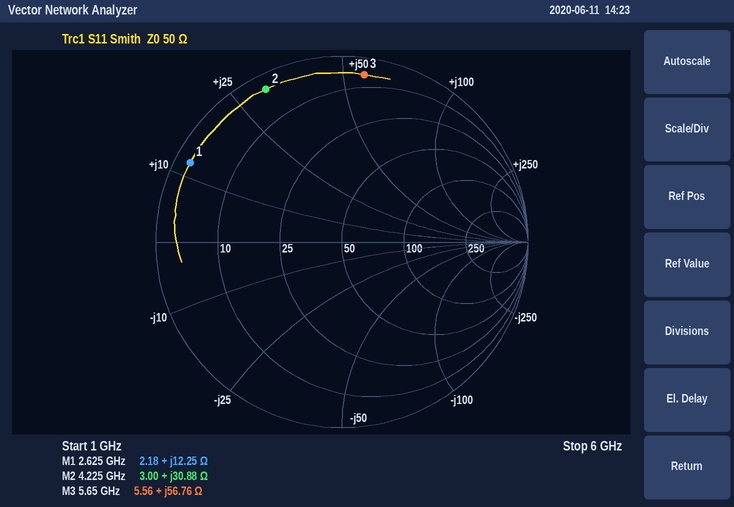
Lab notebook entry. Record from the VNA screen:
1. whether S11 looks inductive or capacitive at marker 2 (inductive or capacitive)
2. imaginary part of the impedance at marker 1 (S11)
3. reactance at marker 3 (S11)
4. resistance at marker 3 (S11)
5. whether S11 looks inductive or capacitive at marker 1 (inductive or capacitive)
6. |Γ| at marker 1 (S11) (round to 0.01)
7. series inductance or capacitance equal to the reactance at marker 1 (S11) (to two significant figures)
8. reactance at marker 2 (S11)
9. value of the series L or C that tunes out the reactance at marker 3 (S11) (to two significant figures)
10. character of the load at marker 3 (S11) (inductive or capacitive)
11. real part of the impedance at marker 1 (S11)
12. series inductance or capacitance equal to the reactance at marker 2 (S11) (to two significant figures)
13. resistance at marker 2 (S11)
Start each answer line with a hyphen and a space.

- inductive
- +12.25 Ω
- +56.76 Ω
- 5.56 Ω
- inductive
- 0.92
- 740 pH
- +30.88 Ω
- 500 fF
- inductive
- 2.18 Ω
- 1.2 nH
- 3.00 Ω
